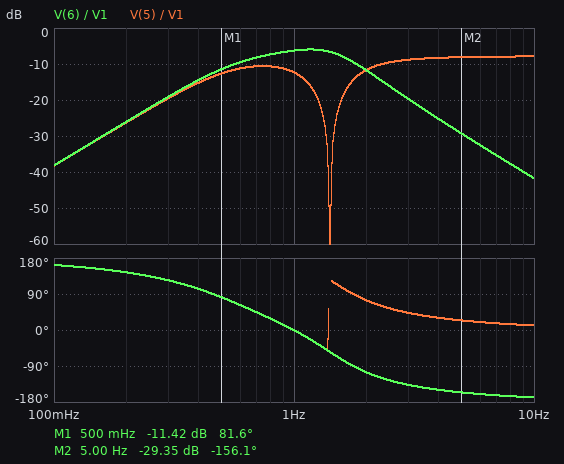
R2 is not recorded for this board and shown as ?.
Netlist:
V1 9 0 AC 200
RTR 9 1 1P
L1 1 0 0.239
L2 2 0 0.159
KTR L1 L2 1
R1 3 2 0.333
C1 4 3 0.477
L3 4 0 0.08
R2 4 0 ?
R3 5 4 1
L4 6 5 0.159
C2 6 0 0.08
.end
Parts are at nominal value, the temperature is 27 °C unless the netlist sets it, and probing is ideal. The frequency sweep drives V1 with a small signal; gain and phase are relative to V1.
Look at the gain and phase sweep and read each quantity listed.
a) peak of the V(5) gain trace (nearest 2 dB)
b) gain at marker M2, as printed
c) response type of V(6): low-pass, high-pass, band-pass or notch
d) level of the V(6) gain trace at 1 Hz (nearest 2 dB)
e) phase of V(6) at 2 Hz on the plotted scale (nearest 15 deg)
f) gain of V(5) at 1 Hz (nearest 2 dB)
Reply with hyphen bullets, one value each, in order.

- -8 dB
- -29.35 dB
- band-pass
- -6 dB
- -105 deg
- -12 dB
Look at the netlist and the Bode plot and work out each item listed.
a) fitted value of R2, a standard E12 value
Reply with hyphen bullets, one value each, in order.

- 0.33 Ω
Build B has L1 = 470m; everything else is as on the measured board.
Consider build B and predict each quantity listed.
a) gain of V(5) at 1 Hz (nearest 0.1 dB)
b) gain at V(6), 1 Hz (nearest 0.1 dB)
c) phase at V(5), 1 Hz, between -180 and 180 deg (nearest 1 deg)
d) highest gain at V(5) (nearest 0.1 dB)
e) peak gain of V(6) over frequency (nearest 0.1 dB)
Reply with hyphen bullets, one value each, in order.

- -15.3 dB
- -9.2 dB
- 0 deg
- -10.8 dB
- -8.9 dB
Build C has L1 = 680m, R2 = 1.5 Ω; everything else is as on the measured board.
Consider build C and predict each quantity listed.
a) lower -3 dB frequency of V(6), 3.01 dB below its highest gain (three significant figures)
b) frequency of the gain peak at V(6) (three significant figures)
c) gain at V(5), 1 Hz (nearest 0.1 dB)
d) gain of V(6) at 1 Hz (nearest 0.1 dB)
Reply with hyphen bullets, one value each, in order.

- 612 mHz
- 933 mHz
- -11.4 dB
- -5.3 dB
